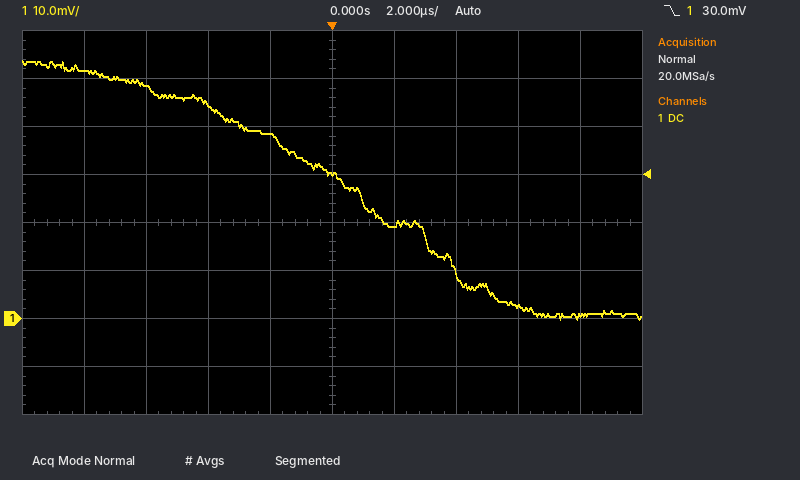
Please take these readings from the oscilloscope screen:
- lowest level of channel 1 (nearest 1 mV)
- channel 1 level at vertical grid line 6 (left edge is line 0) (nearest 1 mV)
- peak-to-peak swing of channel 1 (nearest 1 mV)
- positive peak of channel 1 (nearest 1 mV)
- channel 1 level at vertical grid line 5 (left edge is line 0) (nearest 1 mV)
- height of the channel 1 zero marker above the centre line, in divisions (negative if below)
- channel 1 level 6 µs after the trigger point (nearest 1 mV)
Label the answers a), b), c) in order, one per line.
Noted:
a) 0 mV
b) 20 mV
c) 54 mV
d) 54 mV
e) 30 mV
f) -2.0 div
g) 3 mV
